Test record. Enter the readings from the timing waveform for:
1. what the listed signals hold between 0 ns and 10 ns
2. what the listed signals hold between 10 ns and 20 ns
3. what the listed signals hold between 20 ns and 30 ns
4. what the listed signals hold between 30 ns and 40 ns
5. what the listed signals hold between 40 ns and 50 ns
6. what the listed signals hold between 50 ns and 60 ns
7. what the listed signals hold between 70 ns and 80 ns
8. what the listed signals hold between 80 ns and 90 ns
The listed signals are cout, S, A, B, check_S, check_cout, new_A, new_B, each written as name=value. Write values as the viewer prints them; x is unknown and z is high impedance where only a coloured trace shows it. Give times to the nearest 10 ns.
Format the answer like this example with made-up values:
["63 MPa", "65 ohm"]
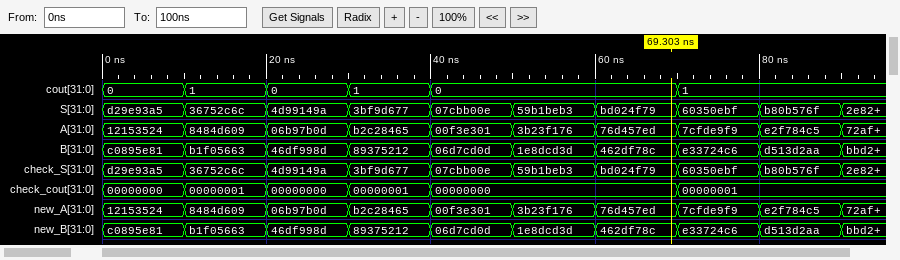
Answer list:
["cout=0, S=d29e93a5, A=12153524, B=c0895e81, check_S=d29e93a5, check_cout=00000000, new_A=12153524, new_B=c0895e81", "cout=1, S=36752c6c, A=8484d609, B=b1f05663, check_S=36752c6c, check_cout=00000001, new_A=8484d609, new_B=b1f05663", "cout=0, S=4d99149a, A=06b97b0d, B=46df998d, check_S=4d99149a, check_cout=00000000, new_A=06b97b0d, new_B=46df998d", "cout=1, S=3bf9d677, A=b2c28465, B=89375212, check_S=3bf9d677, check_cout=00000001, new_A=b2c28465, new_B=89375212", "cout=0, S=07cbb00e, A=00f3e301, B=06d7cd0d, check_S=07cbb00e, check_cout=00000000, new_A=00f3e301, new_B=06d7cd0d", "cout=0, S=59b1beb3, A=3b23f176, B=1e8dcd3d, check_S=59b1beb3, check_cout=00000000, new_A=3b23f176, new_B=1e8dcd3d", "cout=1, S=60350ebf, A=7cfde9f9, B=e33724c6, check_S=60350ebf, check_cout=00000001, new_A=7cfde9f9, new_B=e33724c6", "cout=1, S=b80b576f, A=e2f784c5, B=d513d2aa, check_S=b80b576f, check_cout=00000001, new_A=e2f784c5, new_B=d513d2aa"]
